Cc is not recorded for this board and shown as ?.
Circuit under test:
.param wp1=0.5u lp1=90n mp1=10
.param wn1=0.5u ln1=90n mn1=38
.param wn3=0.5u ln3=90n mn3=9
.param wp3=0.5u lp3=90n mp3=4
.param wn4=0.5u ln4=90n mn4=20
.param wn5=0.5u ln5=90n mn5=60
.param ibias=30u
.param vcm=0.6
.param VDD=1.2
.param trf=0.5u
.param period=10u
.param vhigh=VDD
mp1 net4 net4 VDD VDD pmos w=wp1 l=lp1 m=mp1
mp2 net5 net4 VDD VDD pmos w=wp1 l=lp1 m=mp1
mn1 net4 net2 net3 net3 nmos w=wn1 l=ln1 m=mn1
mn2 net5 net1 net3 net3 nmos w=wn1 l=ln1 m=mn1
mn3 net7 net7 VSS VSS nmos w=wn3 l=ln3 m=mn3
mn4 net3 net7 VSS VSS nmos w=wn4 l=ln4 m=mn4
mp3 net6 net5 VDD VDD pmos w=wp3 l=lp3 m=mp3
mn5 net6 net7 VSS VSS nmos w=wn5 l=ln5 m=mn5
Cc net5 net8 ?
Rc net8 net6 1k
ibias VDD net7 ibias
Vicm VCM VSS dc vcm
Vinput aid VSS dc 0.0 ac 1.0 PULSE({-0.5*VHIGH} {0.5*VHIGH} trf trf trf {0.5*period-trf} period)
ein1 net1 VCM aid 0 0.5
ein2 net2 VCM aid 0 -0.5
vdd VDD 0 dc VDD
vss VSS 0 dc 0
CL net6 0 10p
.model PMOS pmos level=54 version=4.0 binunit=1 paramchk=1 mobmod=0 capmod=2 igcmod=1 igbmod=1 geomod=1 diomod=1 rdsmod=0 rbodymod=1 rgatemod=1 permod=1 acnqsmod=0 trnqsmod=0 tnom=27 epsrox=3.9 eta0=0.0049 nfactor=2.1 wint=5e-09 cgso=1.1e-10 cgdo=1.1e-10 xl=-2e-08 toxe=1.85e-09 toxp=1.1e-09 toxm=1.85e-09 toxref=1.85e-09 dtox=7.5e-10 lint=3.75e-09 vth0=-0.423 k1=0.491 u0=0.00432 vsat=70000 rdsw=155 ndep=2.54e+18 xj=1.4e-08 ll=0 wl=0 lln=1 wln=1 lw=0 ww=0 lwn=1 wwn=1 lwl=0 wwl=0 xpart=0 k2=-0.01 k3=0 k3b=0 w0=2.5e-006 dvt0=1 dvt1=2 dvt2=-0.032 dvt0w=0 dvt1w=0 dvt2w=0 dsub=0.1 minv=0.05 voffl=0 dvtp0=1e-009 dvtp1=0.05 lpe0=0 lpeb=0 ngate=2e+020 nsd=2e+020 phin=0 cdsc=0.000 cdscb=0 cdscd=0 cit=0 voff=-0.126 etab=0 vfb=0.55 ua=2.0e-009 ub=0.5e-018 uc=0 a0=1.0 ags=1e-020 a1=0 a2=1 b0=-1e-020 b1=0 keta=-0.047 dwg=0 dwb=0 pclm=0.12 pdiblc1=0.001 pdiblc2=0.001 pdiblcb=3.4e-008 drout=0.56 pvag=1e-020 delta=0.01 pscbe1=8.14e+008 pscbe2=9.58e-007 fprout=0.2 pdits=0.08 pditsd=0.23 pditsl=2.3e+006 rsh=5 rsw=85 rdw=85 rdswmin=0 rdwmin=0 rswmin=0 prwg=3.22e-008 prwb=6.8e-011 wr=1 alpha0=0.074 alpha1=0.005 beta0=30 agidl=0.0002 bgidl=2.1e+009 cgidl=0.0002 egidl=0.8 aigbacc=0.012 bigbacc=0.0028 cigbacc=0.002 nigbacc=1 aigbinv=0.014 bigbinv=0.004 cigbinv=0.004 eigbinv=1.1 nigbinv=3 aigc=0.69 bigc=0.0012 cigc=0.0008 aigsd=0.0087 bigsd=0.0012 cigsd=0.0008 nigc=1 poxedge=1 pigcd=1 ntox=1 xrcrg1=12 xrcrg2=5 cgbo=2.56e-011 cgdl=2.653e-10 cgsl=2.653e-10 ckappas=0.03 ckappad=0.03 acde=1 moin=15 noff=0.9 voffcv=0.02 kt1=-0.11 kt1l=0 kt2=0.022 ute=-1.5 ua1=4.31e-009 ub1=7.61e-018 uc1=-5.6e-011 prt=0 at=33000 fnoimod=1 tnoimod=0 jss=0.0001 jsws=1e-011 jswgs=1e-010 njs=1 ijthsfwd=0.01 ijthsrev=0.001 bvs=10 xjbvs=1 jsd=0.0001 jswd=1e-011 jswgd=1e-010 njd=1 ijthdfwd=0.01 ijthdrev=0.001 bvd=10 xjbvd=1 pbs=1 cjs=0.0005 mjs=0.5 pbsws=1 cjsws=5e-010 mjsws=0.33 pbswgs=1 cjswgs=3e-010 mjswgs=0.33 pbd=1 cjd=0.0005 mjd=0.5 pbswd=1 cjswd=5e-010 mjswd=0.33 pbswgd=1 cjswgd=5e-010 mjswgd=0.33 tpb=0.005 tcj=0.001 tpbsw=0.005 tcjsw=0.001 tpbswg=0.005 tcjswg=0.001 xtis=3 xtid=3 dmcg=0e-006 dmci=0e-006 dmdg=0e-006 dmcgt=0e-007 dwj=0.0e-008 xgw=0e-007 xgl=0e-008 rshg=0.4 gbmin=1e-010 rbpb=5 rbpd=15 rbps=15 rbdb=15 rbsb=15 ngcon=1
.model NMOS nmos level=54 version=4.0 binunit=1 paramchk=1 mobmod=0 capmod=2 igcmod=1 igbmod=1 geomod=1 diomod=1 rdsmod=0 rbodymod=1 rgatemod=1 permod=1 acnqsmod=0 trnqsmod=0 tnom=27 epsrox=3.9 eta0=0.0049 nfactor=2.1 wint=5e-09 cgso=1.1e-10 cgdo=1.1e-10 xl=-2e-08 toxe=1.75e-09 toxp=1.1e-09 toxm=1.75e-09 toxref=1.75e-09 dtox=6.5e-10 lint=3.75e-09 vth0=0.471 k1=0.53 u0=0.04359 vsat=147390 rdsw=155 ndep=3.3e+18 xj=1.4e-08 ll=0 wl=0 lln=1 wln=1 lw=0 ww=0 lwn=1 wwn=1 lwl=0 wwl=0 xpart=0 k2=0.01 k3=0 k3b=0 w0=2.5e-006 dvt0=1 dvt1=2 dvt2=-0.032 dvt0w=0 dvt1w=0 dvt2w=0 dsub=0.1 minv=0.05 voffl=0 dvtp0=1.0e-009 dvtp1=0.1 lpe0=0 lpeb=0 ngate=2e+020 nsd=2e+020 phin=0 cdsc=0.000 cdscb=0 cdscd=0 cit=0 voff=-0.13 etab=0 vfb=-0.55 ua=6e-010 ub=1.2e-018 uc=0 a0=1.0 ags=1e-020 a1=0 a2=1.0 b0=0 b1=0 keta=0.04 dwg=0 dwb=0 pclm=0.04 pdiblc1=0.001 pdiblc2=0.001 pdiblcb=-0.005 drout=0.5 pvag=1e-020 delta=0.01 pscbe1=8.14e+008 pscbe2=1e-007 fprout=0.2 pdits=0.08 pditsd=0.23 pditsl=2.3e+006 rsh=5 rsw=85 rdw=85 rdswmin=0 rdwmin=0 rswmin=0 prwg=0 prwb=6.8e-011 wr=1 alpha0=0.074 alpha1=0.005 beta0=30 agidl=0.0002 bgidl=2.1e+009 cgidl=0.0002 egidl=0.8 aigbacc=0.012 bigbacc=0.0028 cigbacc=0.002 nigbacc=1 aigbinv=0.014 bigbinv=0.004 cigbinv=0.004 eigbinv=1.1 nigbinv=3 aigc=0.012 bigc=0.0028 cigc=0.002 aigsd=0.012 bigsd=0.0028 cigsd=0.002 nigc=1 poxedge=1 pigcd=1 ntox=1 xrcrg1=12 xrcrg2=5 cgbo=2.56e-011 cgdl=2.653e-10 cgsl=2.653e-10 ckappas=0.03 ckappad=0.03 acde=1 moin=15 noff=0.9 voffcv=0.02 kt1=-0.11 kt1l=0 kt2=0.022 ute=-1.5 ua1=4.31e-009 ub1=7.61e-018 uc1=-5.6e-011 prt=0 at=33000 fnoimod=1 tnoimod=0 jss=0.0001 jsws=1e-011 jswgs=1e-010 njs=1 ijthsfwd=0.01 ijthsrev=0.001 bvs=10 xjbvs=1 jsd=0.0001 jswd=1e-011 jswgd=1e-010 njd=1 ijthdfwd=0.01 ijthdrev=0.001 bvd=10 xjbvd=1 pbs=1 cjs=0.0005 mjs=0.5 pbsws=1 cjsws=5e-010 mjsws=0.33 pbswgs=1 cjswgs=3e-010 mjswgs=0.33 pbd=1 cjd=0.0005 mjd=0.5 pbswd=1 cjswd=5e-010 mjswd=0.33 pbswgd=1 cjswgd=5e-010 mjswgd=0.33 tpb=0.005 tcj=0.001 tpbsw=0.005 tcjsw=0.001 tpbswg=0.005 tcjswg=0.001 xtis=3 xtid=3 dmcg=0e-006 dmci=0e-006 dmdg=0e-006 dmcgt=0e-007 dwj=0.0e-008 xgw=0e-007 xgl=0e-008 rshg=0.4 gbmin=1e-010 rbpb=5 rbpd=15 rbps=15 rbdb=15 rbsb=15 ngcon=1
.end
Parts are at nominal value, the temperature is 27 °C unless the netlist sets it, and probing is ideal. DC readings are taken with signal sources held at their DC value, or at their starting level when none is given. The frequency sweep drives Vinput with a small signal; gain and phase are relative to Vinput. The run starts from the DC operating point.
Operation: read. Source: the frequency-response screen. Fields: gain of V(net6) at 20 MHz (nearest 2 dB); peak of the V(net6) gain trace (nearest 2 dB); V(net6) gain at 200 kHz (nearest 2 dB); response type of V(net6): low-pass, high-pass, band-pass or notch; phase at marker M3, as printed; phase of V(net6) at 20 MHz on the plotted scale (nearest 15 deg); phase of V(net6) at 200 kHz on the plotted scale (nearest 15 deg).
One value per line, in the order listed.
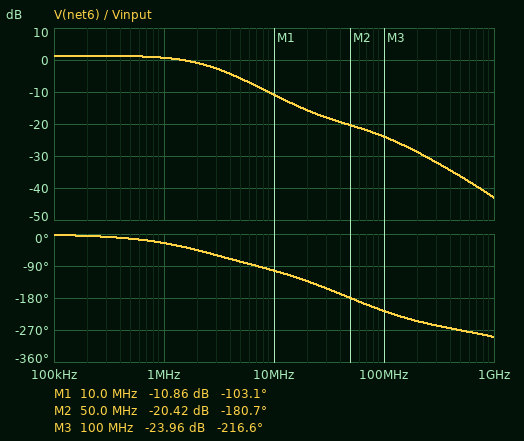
-16 dB
2 dB
2 dB
low-pass
-216.6 deg
-135 deg
0 deg
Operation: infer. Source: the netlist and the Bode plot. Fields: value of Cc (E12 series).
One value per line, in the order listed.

1.2 pF
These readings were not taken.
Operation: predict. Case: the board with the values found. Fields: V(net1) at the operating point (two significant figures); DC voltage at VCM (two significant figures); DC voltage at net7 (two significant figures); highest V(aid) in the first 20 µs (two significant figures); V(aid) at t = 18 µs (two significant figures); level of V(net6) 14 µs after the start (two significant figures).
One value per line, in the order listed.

600 mV
600 mV
430 mV
600 mV
-600 mV
810 mV
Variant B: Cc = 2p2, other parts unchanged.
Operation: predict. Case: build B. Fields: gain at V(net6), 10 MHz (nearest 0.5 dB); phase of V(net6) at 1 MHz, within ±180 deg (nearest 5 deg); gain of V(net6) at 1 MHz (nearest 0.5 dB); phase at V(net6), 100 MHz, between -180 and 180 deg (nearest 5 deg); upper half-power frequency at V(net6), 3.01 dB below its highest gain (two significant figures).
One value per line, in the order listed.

-15.0 dB
-40 deg
-0.5 dB
135 deg
1.3 MHz
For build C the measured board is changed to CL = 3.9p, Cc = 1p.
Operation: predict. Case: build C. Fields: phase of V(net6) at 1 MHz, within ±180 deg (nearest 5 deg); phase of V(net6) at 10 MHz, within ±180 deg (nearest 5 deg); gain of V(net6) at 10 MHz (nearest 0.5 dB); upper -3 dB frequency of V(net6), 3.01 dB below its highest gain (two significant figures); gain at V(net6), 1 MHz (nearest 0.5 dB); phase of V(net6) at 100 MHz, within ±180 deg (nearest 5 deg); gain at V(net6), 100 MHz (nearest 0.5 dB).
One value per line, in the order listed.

-20 deg
-95 deg
-9.5 dB
2.9 MHz
1.0 dB
170 deg
-20.5 dB
